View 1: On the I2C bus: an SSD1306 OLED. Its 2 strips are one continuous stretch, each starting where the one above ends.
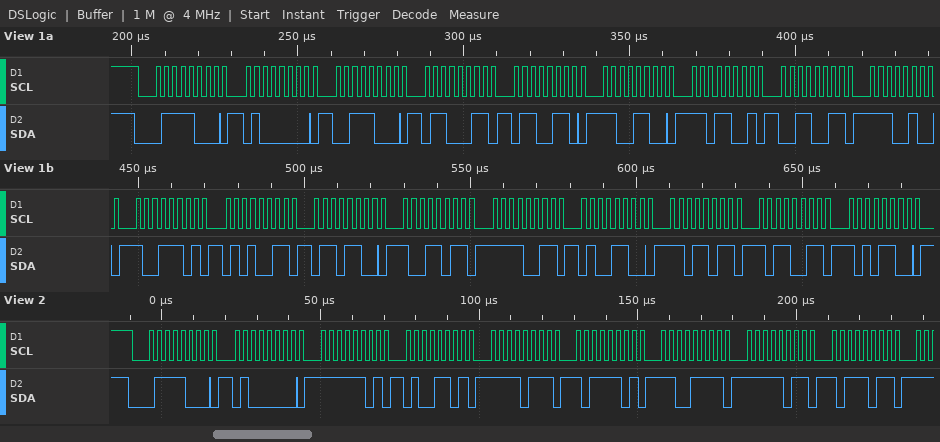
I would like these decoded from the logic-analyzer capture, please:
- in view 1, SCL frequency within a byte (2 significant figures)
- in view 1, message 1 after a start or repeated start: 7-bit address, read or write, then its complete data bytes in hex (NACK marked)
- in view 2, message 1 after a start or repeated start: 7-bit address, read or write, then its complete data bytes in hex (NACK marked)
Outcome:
400 kHz
0x3C write: 40 38 63 66 CC D9 33 E4 9D 53 6C 9B F3 4C DB B3 AC
0x3C write: 40 FD 4D F7 BD CF FB BB
